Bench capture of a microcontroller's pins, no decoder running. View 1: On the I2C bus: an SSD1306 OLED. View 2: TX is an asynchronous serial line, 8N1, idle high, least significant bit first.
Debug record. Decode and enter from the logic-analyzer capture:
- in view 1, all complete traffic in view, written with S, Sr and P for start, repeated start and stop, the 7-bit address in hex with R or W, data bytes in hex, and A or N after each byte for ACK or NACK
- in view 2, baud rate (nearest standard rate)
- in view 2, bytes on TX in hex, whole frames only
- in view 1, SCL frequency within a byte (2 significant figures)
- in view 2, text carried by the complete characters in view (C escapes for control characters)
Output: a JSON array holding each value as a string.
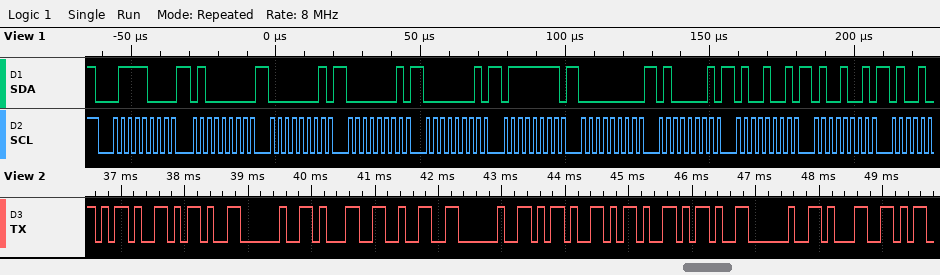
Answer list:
["S 3CW A 40 A 01 A 01 A 01 A 7F A 00 A 41 A 49 A 49 A", "9600 baud", "2D 2D 20 31 32 20 2D 2D 2D 20 31", "400 kHz", "\"-- 12 --- 1\""]
